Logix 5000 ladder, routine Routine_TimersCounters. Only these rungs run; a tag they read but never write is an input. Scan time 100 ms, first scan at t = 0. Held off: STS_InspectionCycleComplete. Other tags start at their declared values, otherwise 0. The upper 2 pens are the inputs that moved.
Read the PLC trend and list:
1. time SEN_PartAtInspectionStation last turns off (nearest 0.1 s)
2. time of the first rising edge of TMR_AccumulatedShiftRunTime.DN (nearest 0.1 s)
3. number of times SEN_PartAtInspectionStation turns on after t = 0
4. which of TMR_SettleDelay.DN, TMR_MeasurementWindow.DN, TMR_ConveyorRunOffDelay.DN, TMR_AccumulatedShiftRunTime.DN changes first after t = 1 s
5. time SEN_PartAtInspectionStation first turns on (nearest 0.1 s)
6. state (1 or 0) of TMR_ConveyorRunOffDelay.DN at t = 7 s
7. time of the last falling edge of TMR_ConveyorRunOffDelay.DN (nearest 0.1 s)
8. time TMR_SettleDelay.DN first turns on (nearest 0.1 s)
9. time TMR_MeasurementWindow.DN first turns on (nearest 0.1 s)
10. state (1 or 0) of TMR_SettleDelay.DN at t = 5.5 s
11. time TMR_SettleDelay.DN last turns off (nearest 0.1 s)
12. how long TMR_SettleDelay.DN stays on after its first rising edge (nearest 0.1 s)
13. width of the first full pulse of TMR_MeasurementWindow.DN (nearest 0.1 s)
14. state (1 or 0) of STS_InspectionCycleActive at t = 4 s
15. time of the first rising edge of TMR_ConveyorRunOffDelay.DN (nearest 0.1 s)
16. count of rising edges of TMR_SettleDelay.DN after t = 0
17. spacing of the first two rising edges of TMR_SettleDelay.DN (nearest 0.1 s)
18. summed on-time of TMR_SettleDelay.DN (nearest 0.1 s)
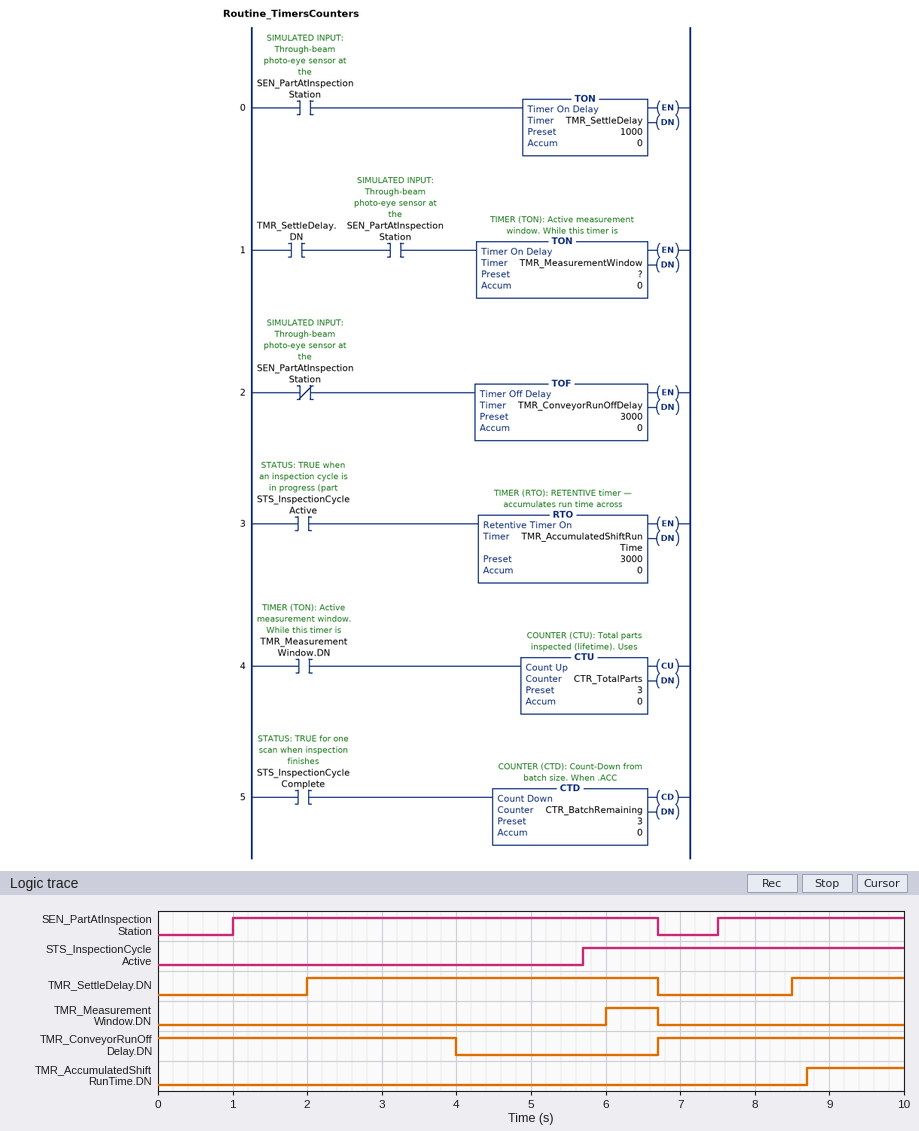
6.7 s
8.7 s
2
TMR_SettleDelay.DN
1.0 s
1
4.0 s
2.0 s
6.0 s
1
6.7 s
4.7 s
0.7 s
0
6.7 s
2
6.5 s
6.2 s
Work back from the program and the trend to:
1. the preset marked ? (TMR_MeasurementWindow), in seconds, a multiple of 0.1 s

4.0 s
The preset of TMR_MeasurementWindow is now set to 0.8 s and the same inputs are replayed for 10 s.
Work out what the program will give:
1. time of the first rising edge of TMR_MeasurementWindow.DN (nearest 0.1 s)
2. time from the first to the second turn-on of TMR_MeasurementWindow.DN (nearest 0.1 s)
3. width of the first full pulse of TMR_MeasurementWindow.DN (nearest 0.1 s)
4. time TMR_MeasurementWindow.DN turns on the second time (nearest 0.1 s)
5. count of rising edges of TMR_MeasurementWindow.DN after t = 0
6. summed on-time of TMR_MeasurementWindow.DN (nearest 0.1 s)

2.8 s
6.5 s
3.9 s
9.3 s
2
4.6 s
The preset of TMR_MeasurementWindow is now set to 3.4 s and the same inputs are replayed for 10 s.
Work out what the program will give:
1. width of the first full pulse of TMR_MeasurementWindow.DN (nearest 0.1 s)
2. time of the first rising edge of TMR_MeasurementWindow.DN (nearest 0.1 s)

1.3 s
5.4 s
